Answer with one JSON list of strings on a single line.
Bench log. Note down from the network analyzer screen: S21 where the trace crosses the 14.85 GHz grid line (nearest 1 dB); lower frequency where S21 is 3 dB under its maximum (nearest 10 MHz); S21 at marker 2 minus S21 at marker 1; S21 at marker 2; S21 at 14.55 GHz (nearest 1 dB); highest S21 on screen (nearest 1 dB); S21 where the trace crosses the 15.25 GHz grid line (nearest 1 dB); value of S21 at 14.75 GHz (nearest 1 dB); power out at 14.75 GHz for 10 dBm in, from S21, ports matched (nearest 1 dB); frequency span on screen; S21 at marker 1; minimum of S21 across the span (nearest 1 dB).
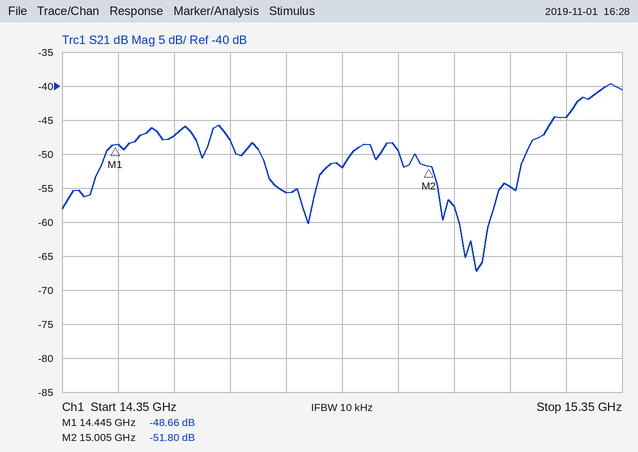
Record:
["-52 dB", "15.27 GHz", "-3.14 dB", "-51.80 dB", "-47 dB", "-40 dB", "-45 dB", "-56 dB", "-46 dBm", "1 GHz", "-48.66 dB", "-67 dB"]
